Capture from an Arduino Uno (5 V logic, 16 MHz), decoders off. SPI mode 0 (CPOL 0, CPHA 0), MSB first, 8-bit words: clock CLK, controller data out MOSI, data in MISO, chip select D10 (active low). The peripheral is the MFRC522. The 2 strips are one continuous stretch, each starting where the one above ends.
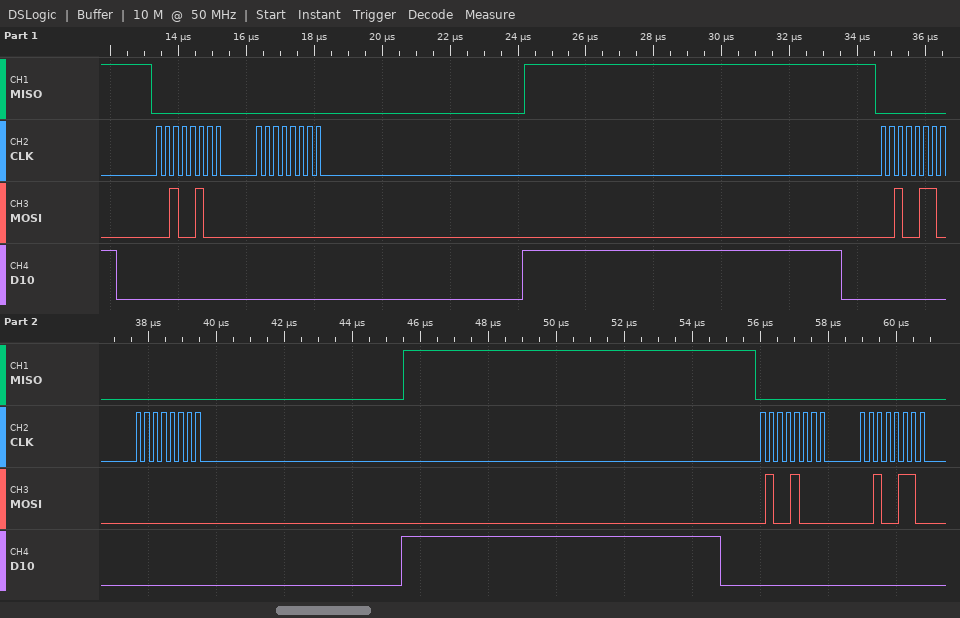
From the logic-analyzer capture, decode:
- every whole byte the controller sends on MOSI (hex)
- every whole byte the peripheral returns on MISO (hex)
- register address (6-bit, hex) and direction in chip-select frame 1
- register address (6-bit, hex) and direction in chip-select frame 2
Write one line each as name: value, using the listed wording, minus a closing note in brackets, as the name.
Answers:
every whole byte the controller sends on MOSI: 0x24 0x00 0x26 0x00 0x48 0x26
every whole byte the peripheral returns on MISO: 0x00 0x00 0x00 0x00 0x00 0x00
register address (6-bit, hex) and direction in chip-select frame 1: 0x12 write
register address (6-bit, hex) and direction in chip-select frame 2: 0x13 write
